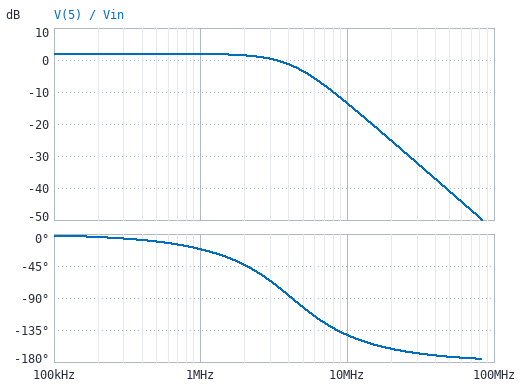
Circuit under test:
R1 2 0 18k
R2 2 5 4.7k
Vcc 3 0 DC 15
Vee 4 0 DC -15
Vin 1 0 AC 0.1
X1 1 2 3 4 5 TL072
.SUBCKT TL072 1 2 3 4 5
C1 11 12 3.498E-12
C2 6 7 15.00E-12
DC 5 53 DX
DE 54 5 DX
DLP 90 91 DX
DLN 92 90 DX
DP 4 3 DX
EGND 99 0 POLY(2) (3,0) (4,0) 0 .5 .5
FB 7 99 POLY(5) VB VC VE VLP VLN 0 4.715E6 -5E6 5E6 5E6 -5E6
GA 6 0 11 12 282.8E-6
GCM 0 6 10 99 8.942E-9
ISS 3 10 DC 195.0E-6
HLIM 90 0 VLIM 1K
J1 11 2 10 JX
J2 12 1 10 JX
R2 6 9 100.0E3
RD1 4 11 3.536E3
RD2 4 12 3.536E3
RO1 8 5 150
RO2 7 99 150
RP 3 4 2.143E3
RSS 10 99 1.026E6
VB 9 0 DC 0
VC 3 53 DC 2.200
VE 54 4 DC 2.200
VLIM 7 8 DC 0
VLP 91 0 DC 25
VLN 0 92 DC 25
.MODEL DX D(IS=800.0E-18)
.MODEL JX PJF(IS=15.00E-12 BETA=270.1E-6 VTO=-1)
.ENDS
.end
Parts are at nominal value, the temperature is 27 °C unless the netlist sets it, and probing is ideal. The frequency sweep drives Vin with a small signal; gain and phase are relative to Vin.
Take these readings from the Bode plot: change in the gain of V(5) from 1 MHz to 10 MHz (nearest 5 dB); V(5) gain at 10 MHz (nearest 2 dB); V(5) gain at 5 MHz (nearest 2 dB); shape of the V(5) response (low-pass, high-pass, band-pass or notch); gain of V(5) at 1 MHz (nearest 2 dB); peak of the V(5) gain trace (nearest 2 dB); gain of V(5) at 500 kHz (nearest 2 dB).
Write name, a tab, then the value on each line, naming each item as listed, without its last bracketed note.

change in the gain of V(5) from 1 MHz to 10 MHz	-15 dB
V(5) gain at 10 MHz	-14 dB
V(5) gain at 5 MHz	-4 dB
shape of the V(5) response	low-pass
gain of V(5) at 1 MHz	2 dB
peak of the V(5) gain trace	2 dB
gain of V(5) at 500 kHz	2 dB
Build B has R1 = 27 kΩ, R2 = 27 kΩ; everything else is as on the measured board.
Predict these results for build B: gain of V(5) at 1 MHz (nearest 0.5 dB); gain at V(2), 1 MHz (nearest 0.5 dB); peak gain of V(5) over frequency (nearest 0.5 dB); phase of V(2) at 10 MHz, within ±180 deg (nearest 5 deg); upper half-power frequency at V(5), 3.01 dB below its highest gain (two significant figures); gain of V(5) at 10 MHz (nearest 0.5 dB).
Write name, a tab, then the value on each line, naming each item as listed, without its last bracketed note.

gain of V(5) at 1 MHz	5.5 dB
gain at V(2), 1 MHz	-0.5 dB
peak gain of V(5) over frequency	6.0 dB
phase of V(2) at 10 MHz, within ±180 deg	-145 deg
upper half-power frequency at V(5), 3.01 dB below its highest gain	2.2 MHz
gain of V(5) at 10 MHz	-14.0 dB
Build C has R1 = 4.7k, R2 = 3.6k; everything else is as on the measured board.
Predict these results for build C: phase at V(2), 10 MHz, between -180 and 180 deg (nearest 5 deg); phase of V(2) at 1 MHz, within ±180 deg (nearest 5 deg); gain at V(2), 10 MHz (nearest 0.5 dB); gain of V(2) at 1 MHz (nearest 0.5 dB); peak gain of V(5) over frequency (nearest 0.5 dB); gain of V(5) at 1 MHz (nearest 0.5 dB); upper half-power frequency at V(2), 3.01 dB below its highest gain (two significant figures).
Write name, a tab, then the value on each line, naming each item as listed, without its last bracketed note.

phase at V(2), 10 MHz, between -180 and 180 deg	-145 deg
phase of V(2) at 1 MHz, within ±180 deg	-30 deg
gain at V(2), 10 MHz	-19.0 dB
gain of V(2) at 1 MHz	-0.5 dB
peak gain of V(5) over frequency	5.0 dB
gain of V(5) at 1 MHz	4.5 dB
upper half-power frequency at V(2), 3.01 dB below its highest gain	2.6 MHz
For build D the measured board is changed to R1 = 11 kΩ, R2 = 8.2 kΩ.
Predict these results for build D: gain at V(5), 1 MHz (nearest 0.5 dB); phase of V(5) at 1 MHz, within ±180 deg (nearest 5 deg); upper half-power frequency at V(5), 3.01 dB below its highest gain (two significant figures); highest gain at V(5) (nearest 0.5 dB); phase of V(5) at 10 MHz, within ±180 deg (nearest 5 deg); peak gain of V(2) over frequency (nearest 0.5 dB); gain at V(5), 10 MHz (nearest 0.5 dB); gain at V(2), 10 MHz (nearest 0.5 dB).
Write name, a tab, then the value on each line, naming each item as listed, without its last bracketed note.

gain at V(5), 1 MHz	4.5 dB
phase of V(5) at 1 MHz, within ±180 deg	-30 deg
upper half-power frequency at V(5), 3.01 dB below its highest gain	2.6 MHz
highest gain at V(5)	5.0 dB
phase of V(5) at 10 MHz, within ±180 deg	-145 deg
peak gain of V(2) over frequency	0 dB
gain at V(5), 10 MHz	-14.0 dB
gain at V(2), 10 MHz	-18.5 dB
